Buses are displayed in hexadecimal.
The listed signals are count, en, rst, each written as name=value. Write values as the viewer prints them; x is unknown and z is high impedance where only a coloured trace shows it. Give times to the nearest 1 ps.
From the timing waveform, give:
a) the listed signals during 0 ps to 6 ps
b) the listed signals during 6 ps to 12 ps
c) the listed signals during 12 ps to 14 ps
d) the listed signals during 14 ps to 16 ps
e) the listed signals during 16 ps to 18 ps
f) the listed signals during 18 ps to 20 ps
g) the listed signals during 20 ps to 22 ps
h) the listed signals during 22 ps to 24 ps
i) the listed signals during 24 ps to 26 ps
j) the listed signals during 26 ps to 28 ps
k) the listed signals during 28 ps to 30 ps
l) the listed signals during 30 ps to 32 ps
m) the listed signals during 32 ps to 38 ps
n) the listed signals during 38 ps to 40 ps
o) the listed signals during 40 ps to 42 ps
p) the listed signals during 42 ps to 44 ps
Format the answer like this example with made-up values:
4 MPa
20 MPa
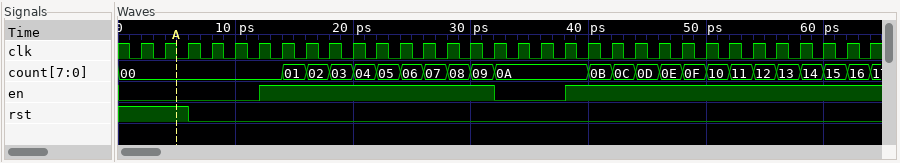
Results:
count=00, en=0, rst=1
count=00, en=0, rst=0
count=00, en=1, rst=0
count=01, en=1, rst=0
count=02, en=1, rst=0
count=03, en=1, rst=0
count=04, en=1, rst=0
count=05, en=1, rst=0
count=06, en=1, rst=0
count=07, en=1, rst=0
count=08, en=1, rst=0
count=09, en=1, rst=0
count=0A, en=0, rst=0
count=0A, en=1, rst=0
count=0B, en=1, rst=0
count=0C, en=1, rst=0
